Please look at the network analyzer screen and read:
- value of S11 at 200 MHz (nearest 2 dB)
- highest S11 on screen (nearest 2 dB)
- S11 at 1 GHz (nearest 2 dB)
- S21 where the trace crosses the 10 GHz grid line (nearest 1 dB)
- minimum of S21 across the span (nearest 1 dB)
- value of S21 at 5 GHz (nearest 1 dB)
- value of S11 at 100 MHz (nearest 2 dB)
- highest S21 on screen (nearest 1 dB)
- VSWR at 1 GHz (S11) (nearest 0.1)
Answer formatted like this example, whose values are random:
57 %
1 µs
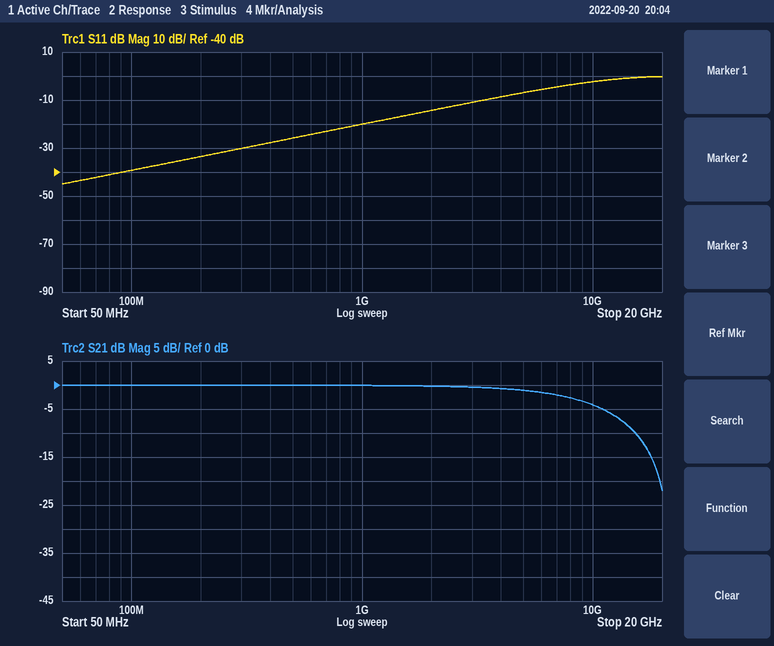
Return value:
-34 dB
0 dB
-20 dB
-4 dB
-22 dB
-1 dB
-40 dB
0 dB
1.2
